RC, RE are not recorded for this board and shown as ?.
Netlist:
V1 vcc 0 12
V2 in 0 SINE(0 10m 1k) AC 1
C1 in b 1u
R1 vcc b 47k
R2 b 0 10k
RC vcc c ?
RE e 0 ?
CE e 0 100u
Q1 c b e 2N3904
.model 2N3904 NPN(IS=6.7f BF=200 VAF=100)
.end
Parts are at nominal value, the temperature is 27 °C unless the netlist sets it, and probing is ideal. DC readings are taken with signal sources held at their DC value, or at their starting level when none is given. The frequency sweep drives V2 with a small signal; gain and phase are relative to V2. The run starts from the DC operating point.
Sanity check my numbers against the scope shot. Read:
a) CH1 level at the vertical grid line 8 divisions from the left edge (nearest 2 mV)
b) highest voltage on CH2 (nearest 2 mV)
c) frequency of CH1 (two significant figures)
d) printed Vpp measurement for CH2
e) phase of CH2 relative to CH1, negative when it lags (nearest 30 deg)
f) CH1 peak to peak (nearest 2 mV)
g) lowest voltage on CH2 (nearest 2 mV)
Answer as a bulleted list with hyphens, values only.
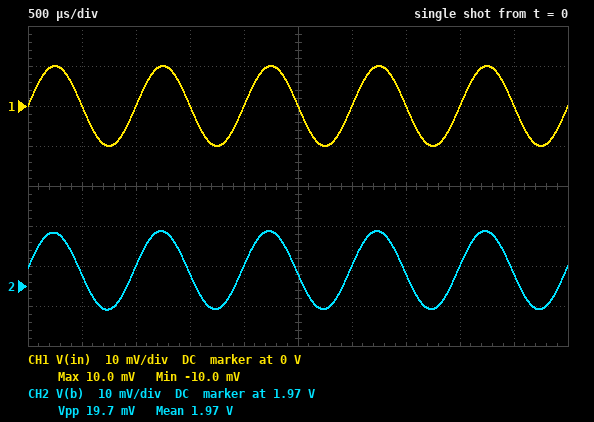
- 0 V
- 1.984 V
- 1.0 kHz
- 19.7 mV
- 0 deg
- 20 mV
- 1.964 V
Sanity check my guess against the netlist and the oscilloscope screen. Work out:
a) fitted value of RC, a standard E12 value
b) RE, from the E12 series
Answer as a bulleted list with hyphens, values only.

- 2.2 kΩ
- 390 Ω
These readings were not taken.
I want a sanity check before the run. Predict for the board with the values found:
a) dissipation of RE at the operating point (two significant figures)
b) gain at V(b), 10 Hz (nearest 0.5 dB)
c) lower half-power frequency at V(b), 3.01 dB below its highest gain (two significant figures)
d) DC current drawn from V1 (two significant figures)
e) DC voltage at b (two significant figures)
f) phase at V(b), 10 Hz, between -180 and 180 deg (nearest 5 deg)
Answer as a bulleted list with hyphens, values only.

- 4.2 mW
- -8.5 dB
- 120 Hz
- 3.5 mA
- 2.0 V
- 55 deg
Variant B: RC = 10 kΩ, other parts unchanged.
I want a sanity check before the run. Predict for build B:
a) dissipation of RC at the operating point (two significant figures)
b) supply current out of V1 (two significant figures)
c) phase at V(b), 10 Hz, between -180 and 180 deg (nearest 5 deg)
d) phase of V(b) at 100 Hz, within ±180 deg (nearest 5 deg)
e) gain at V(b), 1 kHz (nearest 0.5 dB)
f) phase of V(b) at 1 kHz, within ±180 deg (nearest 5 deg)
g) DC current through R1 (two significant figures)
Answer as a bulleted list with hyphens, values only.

- 13 mW
- 1.4 mA
- 35 deg
- 65 deg
- -13.0 dB
- 75 deg
- 230 µA
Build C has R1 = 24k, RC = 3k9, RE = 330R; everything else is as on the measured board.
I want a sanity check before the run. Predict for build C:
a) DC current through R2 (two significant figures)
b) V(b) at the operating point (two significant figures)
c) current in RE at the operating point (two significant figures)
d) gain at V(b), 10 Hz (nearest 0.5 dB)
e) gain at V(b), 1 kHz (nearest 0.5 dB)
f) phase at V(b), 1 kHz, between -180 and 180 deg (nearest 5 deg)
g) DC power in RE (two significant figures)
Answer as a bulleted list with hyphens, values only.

- 170 µA
- 1.7 V
- 3.1 mA
- -40.5 dB
- -20.0 dB
- 80 deg
- 3.1 mW
